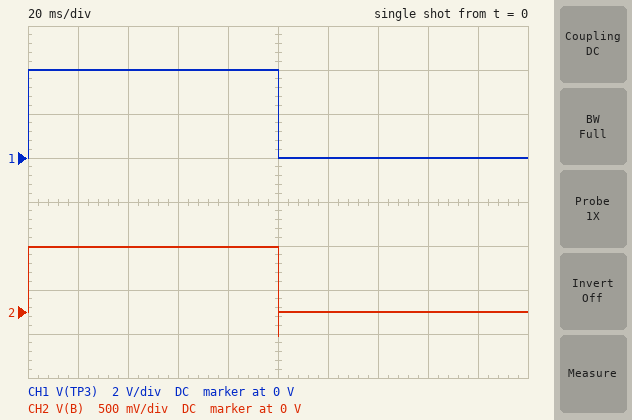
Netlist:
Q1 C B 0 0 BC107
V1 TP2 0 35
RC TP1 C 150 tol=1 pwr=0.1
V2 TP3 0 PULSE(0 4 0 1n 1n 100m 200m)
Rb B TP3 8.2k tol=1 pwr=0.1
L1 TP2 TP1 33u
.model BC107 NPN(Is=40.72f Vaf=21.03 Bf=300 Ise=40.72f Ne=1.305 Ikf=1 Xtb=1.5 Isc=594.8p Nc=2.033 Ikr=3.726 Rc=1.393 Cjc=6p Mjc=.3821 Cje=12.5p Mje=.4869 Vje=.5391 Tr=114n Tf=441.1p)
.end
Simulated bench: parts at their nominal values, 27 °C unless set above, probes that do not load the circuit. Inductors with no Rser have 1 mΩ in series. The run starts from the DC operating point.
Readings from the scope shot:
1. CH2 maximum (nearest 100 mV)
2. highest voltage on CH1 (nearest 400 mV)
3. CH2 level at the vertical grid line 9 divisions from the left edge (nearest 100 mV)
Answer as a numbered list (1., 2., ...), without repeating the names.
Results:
1. 700 mV
2. 4.0 V
3. 0 V
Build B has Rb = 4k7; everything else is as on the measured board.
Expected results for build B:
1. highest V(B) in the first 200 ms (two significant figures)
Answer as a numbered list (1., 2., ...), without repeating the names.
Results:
1. 750 mV
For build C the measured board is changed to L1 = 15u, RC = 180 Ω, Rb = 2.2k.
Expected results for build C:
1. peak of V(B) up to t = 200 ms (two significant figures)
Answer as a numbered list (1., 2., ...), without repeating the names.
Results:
1. 760 mV
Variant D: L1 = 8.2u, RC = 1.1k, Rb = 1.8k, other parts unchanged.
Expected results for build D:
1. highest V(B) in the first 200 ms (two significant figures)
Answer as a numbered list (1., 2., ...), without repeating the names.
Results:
1. 710 mV
